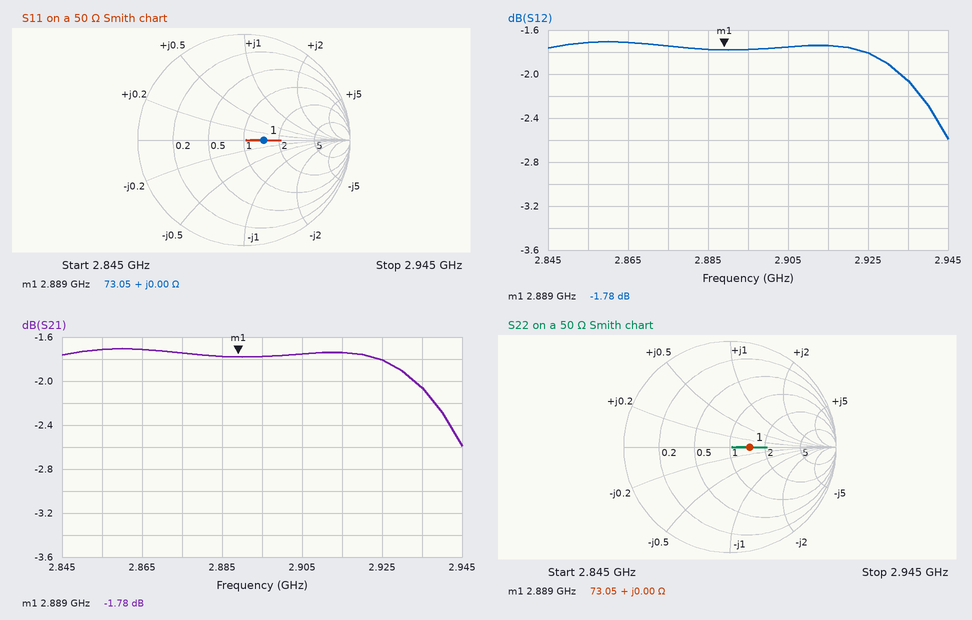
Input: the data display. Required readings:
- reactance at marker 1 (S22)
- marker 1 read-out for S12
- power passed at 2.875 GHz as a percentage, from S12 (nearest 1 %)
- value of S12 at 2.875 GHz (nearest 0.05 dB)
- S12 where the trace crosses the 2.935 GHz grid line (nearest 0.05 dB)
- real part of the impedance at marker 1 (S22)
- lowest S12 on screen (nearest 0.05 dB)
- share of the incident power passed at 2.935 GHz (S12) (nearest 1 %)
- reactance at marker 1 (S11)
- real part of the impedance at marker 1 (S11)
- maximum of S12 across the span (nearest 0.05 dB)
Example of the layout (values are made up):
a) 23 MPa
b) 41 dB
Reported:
a) +0.00 Ω
b) -1.78 dB
c) 67 %
d) -1.75 dB
e) -2.05 dB
f) 73.05 Ω
g) -2.60 dB
h) 62 %
i) +0.00 Ω
j) 73.05 Ω
k) -1.70 dB
